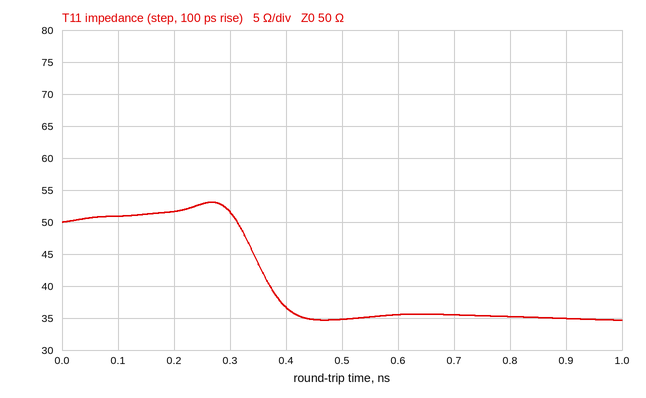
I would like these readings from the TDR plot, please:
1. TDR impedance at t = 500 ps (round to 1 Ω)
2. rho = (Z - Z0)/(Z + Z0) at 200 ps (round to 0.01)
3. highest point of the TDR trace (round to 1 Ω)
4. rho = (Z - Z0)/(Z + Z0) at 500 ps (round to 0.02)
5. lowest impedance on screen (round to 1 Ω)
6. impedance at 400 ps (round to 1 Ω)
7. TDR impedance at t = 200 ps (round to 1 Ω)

35 Ω
+0.02
53 Ω
-0.18
35 Ω
37 Ω
52 Ω
